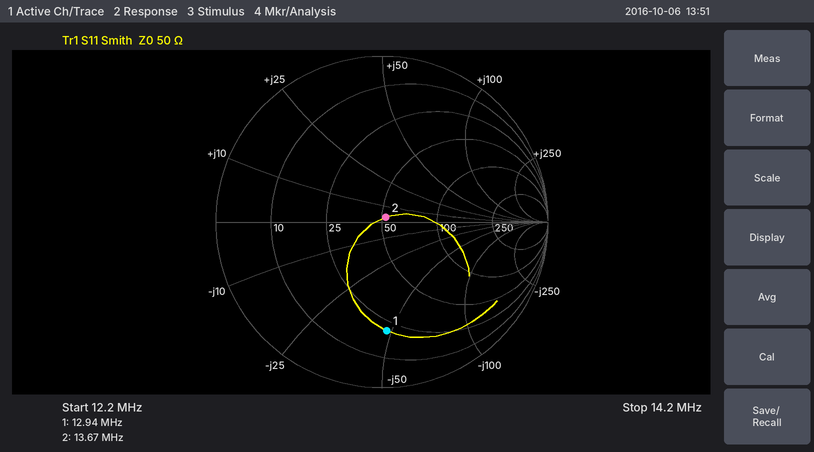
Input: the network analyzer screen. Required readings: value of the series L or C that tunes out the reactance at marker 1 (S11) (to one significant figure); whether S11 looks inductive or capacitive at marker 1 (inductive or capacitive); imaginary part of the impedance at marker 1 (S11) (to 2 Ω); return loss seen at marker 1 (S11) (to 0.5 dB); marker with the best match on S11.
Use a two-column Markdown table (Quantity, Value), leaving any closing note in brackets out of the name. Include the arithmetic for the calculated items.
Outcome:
| Quantity | Value |
|---|---|
| value of the series L or C that tunes out the reactance at marker 1 (S11) | L = 48 Ω/(2π × 12.94 MHz) ≈ 590 nH, so 600 nH to one significant figure |
| whether S11 looks inductive or capacitive at marker 1 | capacitive |
| imaginary part of the impedance at marker 1 (S11) | -48 Ω |
| return loss seen at marker 1 (S11) | 3.5 dB |
| marker with the best match on S11 | marker 2 |
